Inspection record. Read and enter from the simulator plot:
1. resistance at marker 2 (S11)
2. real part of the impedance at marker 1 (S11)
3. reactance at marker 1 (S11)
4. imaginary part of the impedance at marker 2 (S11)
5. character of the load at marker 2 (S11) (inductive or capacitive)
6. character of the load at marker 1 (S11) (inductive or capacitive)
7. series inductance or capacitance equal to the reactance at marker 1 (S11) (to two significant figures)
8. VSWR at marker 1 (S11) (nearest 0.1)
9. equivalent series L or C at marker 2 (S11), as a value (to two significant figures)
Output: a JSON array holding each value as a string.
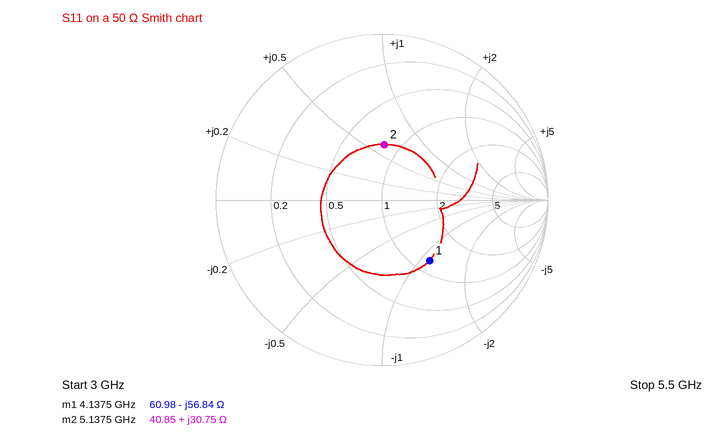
["40.85 Ω", "60.98 Ω", "-56.84 Ω", "+30.75 Ω", "inductive", "capacitive", "680 fF", "2.7", "950 pH"]
